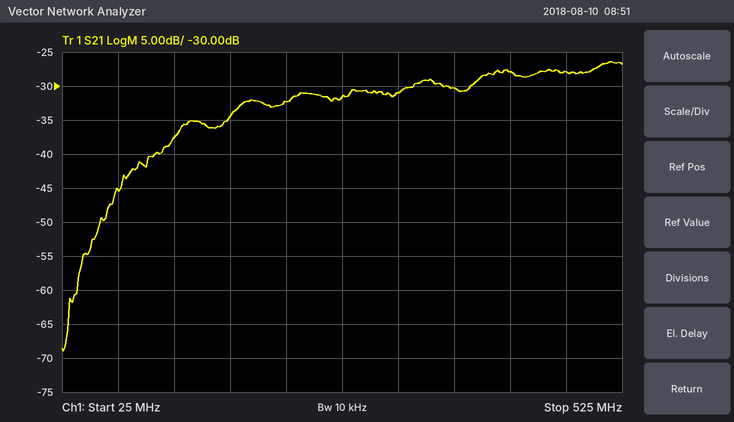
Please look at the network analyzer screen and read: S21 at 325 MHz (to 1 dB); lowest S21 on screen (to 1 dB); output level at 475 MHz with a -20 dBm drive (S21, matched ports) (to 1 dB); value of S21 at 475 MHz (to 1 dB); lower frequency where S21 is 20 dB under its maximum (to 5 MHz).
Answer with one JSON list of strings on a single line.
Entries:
["-31 dB", "-69 dB", "-48 dBm", "-28 dB", "70 MHz"]
